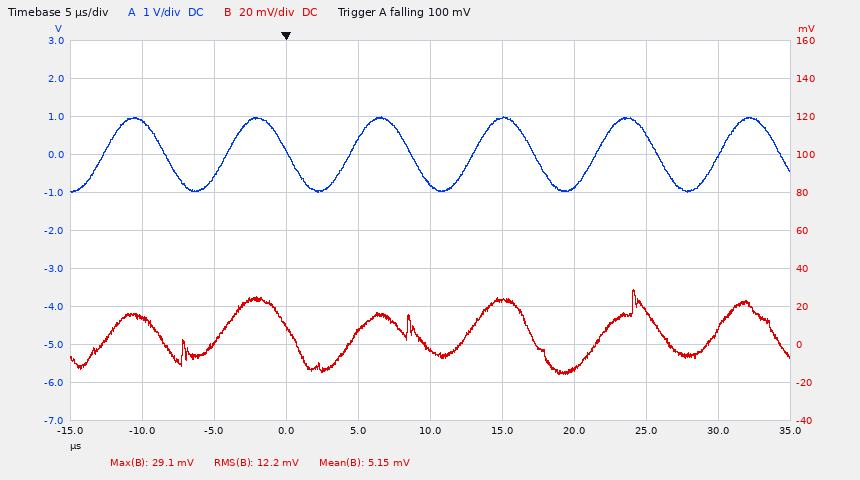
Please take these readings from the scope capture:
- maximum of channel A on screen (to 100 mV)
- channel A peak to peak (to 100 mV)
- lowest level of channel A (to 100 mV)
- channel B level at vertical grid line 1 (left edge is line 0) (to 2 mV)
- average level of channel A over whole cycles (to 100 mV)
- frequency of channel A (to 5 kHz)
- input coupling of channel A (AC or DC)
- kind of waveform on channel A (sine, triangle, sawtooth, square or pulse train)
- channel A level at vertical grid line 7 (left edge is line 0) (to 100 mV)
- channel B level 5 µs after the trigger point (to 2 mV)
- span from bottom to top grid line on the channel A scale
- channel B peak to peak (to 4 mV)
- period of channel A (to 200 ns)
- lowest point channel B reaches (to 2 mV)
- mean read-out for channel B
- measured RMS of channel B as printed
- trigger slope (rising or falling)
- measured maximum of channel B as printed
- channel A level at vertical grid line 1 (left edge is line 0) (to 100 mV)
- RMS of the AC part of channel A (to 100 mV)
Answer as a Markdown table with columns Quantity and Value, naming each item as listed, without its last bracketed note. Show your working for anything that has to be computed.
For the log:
| Quantity | Value |
|---|---|
| maximum of channel A on screen | 1.0 V |
| channel A peak to peak | 1.0 V − (-1.0 V) = 2.0 V |
| lowest level of channel A | -1.0 V |
| channel B level at vertical grid line 1 (left edge is line 0) | 14 mV |
| average level of channel A over whole cycles | (1.0 V + (-1.0 V)) / 2 ≈ 0.0 V |
| frequency of channel A | 1 / 8.6 µs ≈ 116 kHz, so 115 kHz to the nearest 5 kHz |
| input coupling of channel A | DC |
| kind of waveform on channel A | sine |
| channel A level at vertical grid line 7 (left edge is line 0) | -900 mV |
| channel B level 5 µs after the trigger point | 8 mV |
| span from bottom to top grid line on the channel A scale | 10 V |
| channel B peak to peak | 44 mV |
| period of channel A | 8.6 µs |
| lowest point channel B reaches | -16 mV |
| mean read-out for channel B | 5.15 mV |
| measured RMS of channel B as printed | 12.2 mV |
| trigger slope | falling |
| measured maximum of channel B as printed | 29.1 mV |
| channel A level at vertical grid line 1 (left edge is line 0) | 900 mV |
| RMS of the AC part of channel A | 2.0 V / (2√2) ≈ 707 mV, so 700 mV to the nearest 100 mV |
